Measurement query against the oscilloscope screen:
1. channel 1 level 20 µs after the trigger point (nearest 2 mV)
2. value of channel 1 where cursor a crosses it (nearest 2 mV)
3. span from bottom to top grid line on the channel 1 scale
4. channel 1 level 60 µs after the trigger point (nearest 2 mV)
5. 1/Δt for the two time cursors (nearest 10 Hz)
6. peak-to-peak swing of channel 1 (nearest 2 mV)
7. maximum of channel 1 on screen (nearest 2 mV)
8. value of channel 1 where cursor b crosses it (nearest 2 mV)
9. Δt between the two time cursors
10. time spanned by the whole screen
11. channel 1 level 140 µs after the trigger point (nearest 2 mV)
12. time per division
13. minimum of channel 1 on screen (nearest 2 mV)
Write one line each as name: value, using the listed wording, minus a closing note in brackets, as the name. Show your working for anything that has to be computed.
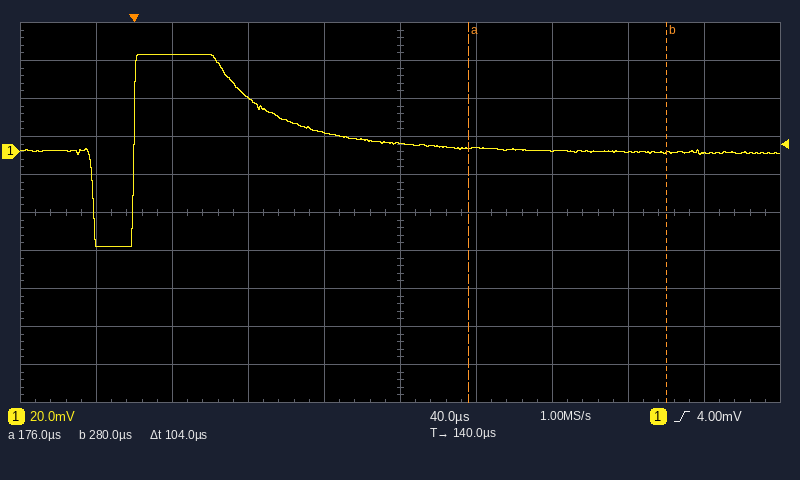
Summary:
channel 1 level 20 µs after the trigger point: 52 mV
value of channel 1 where cursor a crosses it: 2 mV
span from bottom to top grid line on the channel 1 scale: 200 mV
channel 1 level 60 µs after the trigger point: 28 mV
1/Δt for the two time cursors: 1 / 104 µs ≈ 9.62 kHz
peak-to-peak swing of channel 1: 52 mV − (-50 mV) = 102 mV
maximum of channel 1 on screen: 52 mV
value of channel 1 where cursor b crosses it: 0 mV
Δt between the two time cursors: 104 µs
time spanned by the whole screen: 400 µs
channel 1 level 140 µs after the trigger point: 4 mV
time per division: 40 µs
minimum of channel 1 on screen: -50 mV
